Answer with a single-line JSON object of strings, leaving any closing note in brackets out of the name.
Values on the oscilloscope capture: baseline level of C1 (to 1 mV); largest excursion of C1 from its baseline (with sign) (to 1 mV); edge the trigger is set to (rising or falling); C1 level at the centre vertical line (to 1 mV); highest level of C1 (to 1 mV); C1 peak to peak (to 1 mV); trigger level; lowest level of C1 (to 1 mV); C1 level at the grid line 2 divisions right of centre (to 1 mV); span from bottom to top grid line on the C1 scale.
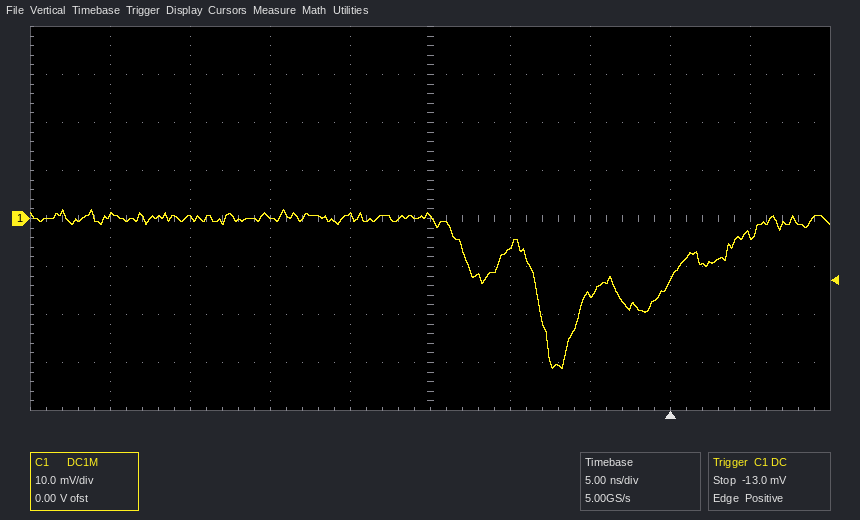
{"baseline level of C1": "0 mV", "largest excursion of C1 from its baseline (with sign)": "-31 mV", "edge the trigger is set to": "rising", "C1 level at the centre vertical line": "0 mV", "highest level of C1": "2 mV", "C1 peak to peak": "33 mV", "trigger level": "-13.0 mV", "lowest level of C1": "-31 mV", "C1 level at the grid line 2 divisions right of centre": "-16 mV", "span from bottom to top grid line on the C1 scale": "80 mV"}
